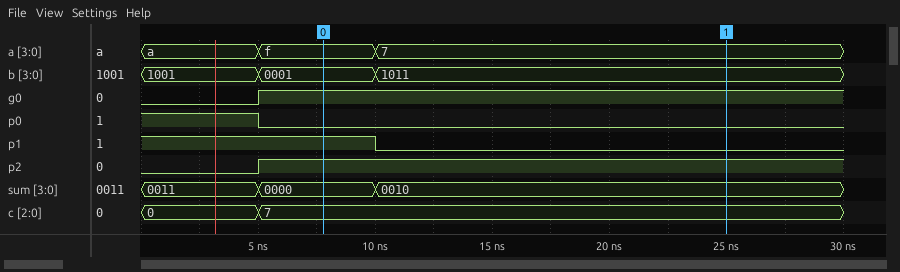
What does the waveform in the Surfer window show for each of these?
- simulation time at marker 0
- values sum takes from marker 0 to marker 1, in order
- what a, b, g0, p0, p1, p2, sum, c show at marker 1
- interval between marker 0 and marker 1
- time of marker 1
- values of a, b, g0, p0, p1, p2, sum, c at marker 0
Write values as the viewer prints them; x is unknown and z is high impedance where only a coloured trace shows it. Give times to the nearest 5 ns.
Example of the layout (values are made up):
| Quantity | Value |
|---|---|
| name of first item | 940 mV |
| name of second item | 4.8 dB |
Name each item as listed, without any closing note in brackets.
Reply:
| Quantity | Value |
|---|---|
| simulation time at marker 0 | 10 ns |
| values sum takes from marker 0 to marker 1, in order | 0000, 0010 |
| what a, b, g0, p0, p1, p2, sum, c show at marker 1 | a=7, b=1011, g0=1, p0=0, p1=0, p2=1, sum=0010, c=7 |
| interval between marker 0 and marker 1 | 15 ns |
| time of marker 1 | 25 ns |
| values of a, b, g0, p0, p1, p2, sum, c at marker 0 | a=f, b=0001, g0=1, p0=0, p1=1, p2=1, sum=0000, c=7 |
